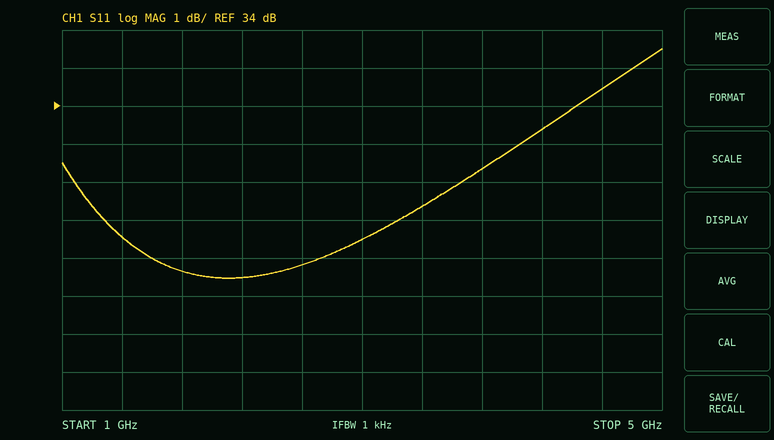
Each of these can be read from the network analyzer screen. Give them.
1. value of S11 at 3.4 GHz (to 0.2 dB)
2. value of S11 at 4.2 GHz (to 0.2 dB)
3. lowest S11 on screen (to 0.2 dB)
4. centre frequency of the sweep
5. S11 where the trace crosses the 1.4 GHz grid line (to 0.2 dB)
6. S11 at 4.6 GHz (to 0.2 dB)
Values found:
31.4 dB
33.4 dB
29.4 dB
3 GHz
30.6 dB
34.4 dB
